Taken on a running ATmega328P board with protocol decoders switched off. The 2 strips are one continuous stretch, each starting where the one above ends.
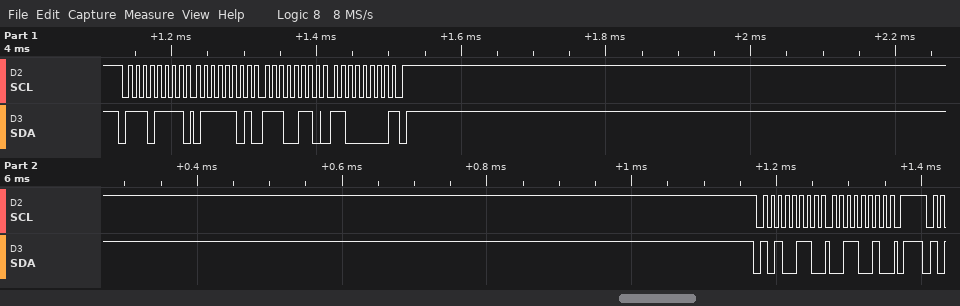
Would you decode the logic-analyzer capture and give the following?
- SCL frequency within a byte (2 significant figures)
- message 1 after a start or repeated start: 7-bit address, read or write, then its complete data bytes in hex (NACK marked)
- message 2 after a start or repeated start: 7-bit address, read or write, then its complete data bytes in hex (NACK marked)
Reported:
100 kHz
0x77 read: 7D E6 C0 NACK
0x53 write: 32
